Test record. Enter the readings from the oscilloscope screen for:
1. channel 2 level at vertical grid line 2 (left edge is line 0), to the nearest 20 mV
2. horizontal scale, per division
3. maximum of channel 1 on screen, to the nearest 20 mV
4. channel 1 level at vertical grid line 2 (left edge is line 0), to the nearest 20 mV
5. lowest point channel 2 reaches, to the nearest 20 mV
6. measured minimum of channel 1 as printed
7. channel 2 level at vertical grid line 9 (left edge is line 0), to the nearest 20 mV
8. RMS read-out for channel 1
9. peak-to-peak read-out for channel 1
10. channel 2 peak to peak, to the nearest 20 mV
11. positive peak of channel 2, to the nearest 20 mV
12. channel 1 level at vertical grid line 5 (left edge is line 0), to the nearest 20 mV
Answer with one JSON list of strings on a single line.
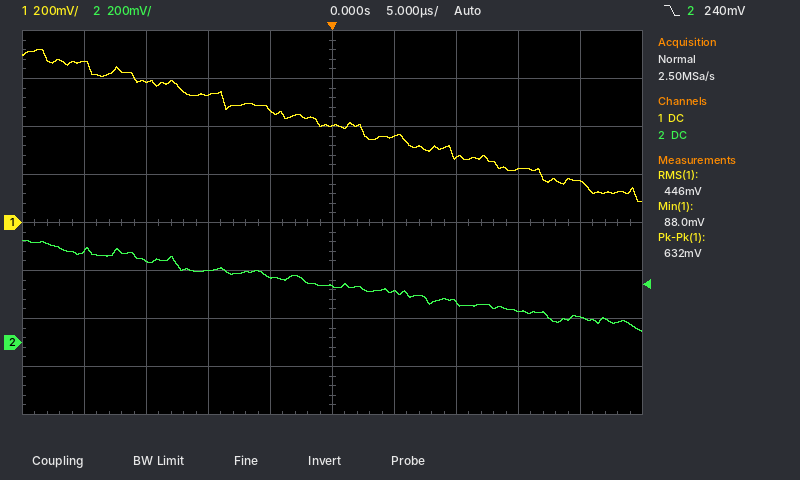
["340 mV", "5 µs", "720 mV", "580 mV", "40 mV", "88.0 mV", "100 mV", "446 mV", "632 mV", "380 mV", "420 mV", "400 mV"]
